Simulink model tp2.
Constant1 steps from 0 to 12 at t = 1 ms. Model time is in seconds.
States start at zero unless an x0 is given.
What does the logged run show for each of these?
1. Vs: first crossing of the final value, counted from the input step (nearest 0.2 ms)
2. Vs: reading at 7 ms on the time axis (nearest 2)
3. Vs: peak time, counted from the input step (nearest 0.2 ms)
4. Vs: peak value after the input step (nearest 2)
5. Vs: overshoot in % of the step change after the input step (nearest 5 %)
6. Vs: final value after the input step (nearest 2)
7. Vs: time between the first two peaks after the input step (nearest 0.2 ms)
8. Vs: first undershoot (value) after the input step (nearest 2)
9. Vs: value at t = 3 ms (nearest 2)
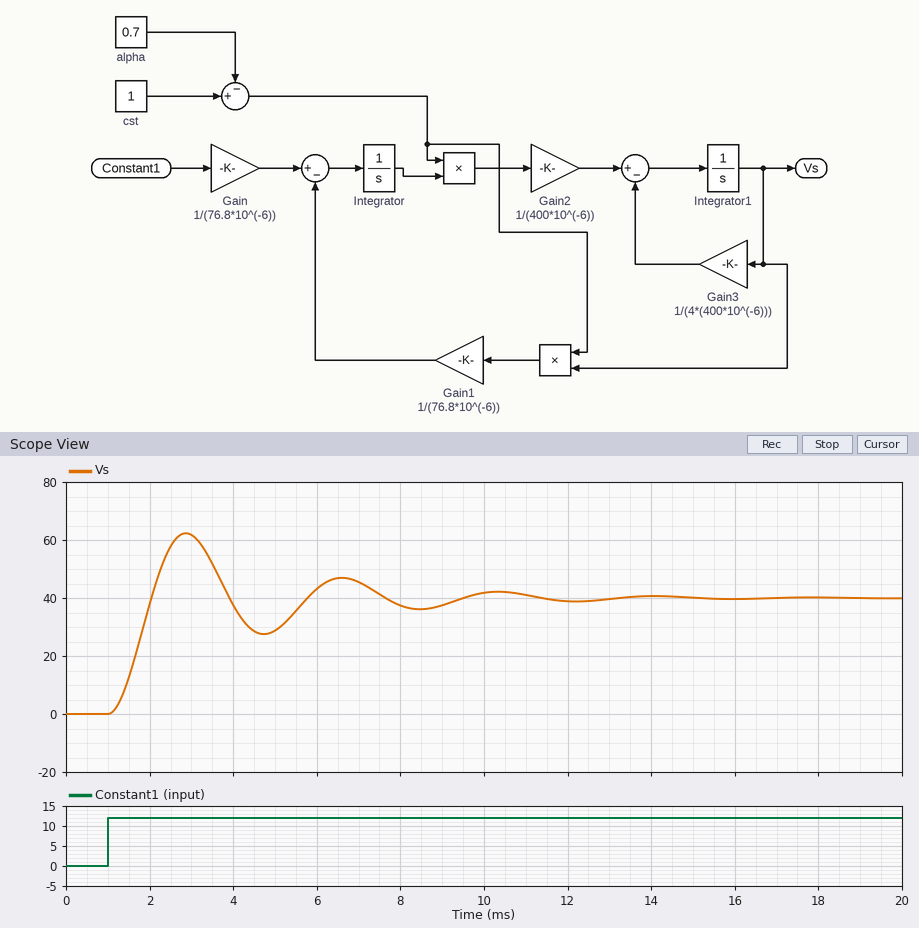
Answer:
1.0 ms
46
1.8 ms
62
55 %
40
3.8 ms
28
62
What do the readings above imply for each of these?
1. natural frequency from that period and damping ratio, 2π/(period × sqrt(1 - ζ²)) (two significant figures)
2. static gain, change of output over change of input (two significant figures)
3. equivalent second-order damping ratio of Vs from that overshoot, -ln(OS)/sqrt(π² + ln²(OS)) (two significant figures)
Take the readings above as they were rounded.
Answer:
1.7 rad/ms
3.3
0.19
